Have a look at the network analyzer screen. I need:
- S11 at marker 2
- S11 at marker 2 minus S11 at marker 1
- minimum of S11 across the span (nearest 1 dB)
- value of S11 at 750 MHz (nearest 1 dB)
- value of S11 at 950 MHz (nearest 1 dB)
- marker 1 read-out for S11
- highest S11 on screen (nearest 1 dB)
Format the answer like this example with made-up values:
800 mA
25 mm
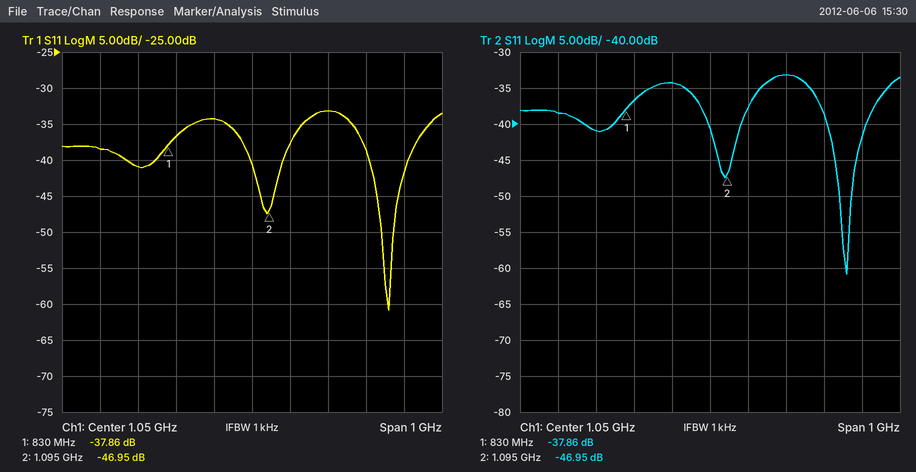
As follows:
-46.95 dB
-9.09 dB
-61 dB
-41 dB
-34 dB
-37.86 dB
-33 dB
